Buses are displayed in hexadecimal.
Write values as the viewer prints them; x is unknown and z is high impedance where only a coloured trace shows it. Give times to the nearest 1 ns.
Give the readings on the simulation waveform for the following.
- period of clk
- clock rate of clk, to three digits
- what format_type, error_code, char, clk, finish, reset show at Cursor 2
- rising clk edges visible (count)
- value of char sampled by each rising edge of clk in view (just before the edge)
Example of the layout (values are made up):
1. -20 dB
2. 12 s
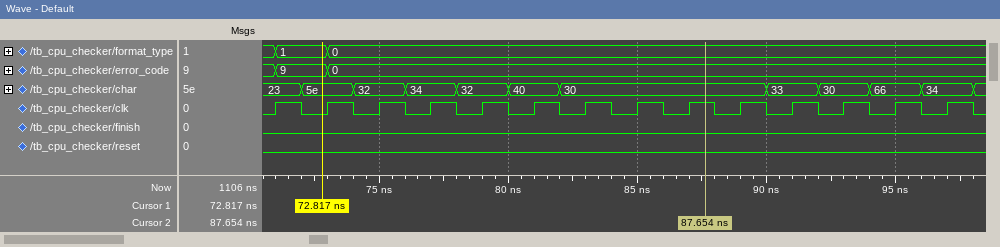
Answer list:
1. 2 ns
2. 500 MHz
3. format_type=0, error_code=0, char=30, clk=1, finish=0, reset=0
4. 14
5. 23, 5e, 32, 34, 32, 40, 30, 30, 30, 30, 33, 30, 66, 34
